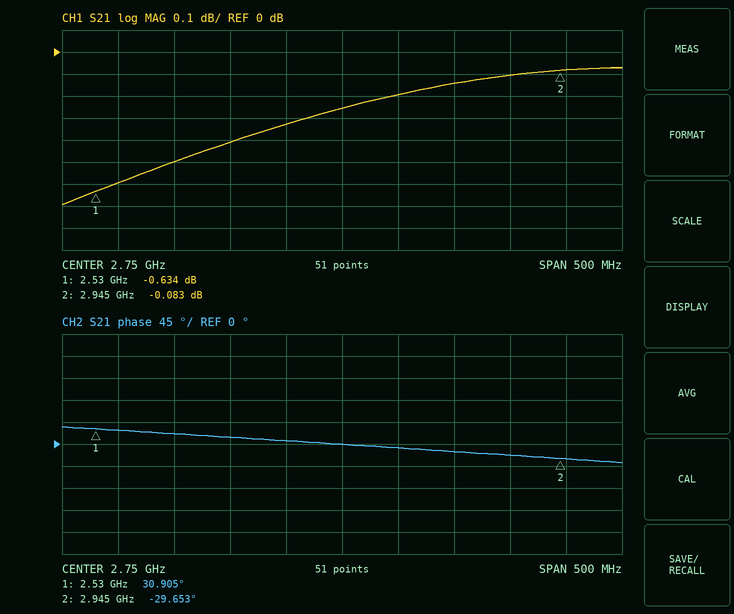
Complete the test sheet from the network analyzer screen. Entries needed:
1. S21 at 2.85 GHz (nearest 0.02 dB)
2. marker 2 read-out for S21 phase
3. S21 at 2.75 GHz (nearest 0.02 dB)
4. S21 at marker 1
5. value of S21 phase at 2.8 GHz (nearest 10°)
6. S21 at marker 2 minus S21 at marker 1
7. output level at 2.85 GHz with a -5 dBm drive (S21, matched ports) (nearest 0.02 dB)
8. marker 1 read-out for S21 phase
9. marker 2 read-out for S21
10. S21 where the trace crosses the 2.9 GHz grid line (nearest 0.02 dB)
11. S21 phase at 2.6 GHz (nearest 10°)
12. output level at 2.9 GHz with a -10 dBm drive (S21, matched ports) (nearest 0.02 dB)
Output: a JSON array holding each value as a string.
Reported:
["-0.14 dB", "-29.653°", "-0.26 dB", "-0.634 dB", "-10°", "0.551 dB", "-5.14 dBm", "30.905°", "-0.083 dB", "-0.10 dB", "20°", "-10.10 dBm"]
